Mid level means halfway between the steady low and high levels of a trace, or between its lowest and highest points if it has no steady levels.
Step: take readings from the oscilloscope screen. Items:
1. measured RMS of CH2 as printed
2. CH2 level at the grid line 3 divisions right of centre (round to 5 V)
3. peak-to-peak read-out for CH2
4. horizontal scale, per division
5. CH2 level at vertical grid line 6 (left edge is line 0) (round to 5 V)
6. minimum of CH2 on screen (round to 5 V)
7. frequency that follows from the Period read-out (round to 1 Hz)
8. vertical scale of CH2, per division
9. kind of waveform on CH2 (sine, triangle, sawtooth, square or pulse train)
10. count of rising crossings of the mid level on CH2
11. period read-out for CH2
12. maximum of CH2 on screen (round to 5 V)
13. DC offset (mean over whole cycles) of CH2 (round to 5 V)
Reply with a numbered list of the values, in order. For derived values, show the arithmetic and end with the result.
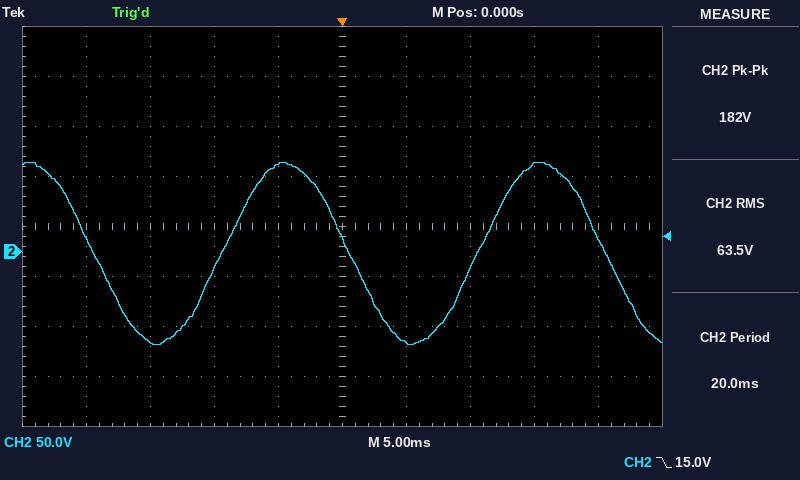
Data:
1. 63.5 V
2. 85 V
3. 182 V
4. 5 ms
5. -90 V
6. -95 V
7. 1 / 20.0 ms ≈ 50 Hz
8. 50 V
9. sine
10. 2
11. 20.0 ms
12. 90 V
13. (90 V + (-95 V)) / 2 ≈ 0 V
